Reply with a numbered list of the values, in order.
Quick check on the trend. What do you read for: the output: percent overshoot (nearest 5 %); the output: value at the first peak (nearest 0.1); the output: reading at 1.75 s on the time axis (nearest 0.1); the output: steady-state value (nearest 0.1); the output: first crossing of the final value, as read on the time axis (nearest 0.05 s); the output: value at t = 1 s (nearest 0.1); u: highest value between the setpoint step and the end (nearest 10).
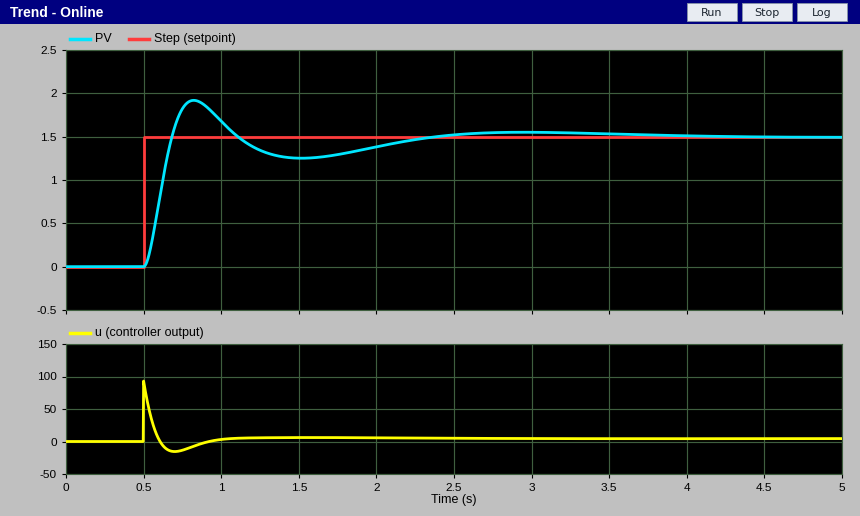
1. 30 %
2. 1.9
3. 1.3
4. 1.5
5. 0.70 s
6. 1.7
7. 90
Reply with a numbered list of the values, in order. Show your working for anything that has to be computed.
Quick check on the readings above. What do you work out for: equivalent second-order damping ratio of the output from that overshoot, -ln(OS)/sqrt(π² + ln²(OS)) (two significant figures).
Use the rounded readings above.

1. ln(0.3) = -1.204; 1.204 / sqrt(9.870 + 1.450) = 0.36
